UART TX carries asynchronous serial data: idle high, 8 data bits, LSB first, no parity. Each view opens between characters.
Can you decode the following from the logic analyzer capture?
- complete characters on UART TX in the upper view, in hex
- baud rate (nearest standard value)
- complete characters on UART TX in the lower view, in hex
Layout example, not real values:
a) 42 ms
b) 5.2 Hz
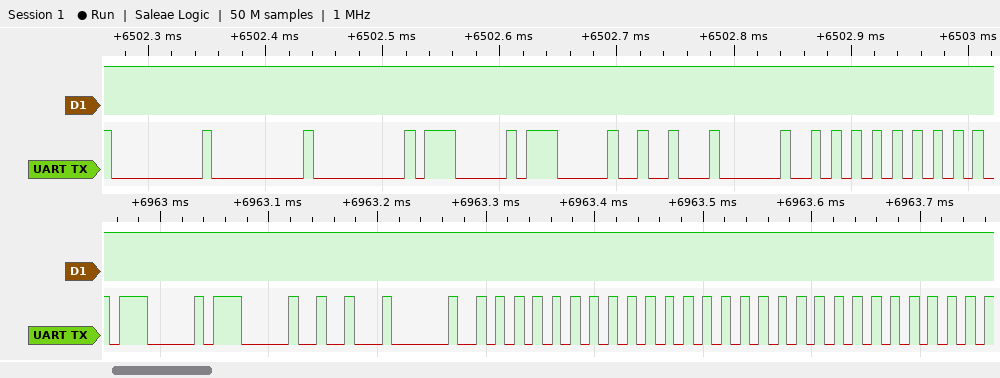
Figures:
a) 00, 00, 00, 07, 07, 12, 20, 55
b) 115200 baud
c) 07, 07, 12, 20, 55, 55, 55, 55, 55
